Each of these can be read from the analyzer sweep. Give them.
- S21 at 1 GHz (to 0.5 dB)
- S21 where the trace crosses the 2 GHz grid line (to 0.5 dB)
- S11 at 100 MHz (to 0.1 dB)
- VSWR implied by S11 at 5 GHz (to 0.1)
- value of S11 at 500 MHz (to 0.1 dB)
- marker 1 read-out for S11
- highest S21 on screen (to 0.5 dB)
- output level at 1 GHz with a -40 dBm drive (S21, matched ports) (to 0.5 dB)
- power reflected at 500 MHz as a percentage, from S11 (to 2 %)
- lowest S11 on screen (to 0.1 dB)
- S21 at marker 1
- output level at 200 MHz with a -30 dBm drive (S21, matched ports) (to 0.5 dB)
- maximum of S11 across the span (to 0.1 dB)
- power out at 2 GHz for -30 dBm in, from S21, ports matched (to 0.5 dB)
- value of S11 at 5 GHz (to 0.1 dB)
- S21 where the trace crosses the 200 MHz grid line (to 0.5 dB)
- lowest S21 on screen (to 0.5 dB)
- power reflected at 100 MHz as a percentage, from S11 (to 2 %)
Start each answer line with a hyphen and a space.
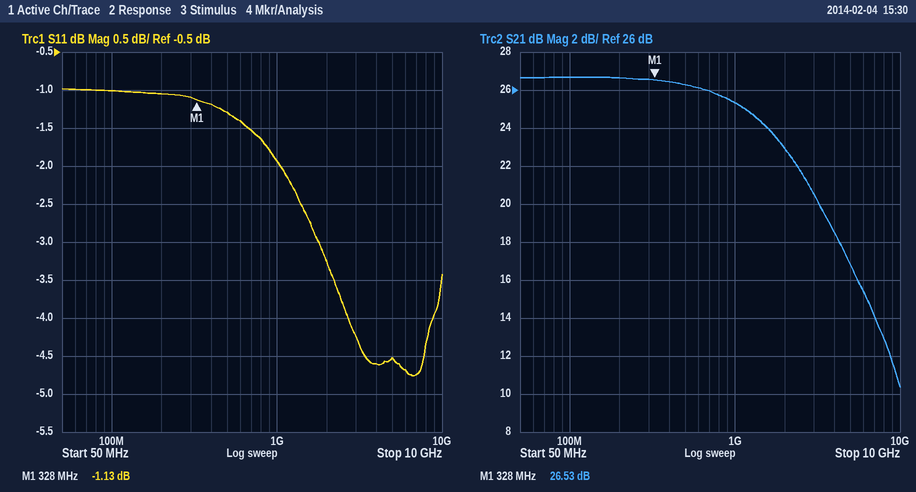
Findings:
- 25.5 dB
- 23.0 dB
- -1.0 dB
- 3.9
- -1.3 dB
- -1.13 dB
- 26.5 dB
- -14.5 dBm
- 74 %
- -4.8 dB
- 26.53 dB
- -3.5 dBm
- -1.0 dB
- -7.0 dBm
- -4.5 dB
- 26.5 dB
- 10.5 dB
- 80 %
